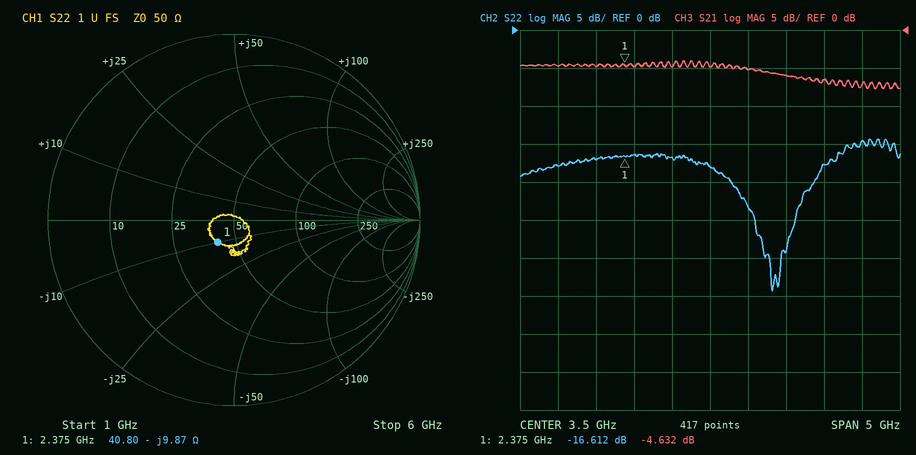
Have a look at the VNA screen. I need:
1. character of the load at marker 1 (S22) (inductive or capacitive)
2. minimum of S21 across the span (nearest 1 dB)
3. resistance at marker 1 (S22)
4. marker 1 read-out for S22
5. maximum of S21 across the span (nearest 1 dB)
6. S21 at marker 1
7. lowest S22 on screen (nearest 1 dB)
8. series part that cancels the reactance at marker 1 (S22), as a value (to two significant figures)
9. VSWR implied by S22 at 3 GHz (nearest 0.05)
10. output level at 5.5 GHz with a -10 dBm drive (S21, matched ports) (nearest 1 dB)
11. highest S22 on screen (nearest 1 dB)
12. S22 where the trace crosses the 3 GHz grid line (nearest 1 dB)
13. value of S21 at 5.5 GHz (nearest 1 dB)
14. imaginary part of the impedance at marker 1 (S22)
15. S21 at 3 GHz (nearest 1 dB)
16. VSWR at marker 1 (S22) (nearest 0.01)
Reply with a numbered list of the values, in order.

1. capacitive
2. -8 dB
3. 40.80 Ω
4. -16.612 dB
5. -4 dB
6. -4.632 dB
7. -34 dB
8. 660 pH
9. 1.35
10. -17 dBm
11. -14 dB
12. -17 dB
13. -7 dB
14. -9.87 Ω
15. -5 dB
16. 1.35
